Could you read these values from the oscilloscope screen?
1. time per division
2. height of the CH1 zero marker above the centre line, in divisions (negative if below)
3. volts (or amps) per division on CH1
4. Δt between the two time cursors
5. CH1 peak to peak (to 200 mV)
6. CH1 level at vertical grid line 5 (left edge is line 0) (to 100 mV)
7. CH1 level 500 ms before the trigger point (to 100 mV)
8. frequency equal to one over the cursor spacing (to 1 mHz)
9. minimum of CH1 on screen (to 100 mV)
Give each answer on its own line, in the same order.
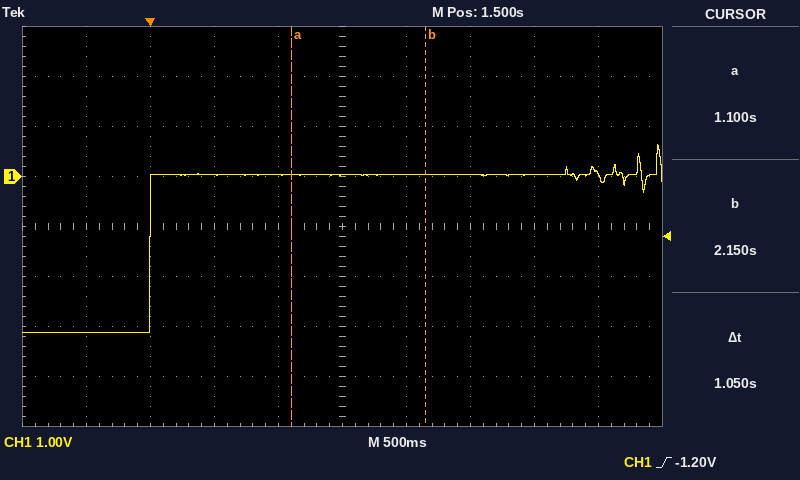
500 ms
+1.0 div
1 V
1.05 s
3.8 V
0.0 V
-3.1 V
952 mHz
-3.1 V
